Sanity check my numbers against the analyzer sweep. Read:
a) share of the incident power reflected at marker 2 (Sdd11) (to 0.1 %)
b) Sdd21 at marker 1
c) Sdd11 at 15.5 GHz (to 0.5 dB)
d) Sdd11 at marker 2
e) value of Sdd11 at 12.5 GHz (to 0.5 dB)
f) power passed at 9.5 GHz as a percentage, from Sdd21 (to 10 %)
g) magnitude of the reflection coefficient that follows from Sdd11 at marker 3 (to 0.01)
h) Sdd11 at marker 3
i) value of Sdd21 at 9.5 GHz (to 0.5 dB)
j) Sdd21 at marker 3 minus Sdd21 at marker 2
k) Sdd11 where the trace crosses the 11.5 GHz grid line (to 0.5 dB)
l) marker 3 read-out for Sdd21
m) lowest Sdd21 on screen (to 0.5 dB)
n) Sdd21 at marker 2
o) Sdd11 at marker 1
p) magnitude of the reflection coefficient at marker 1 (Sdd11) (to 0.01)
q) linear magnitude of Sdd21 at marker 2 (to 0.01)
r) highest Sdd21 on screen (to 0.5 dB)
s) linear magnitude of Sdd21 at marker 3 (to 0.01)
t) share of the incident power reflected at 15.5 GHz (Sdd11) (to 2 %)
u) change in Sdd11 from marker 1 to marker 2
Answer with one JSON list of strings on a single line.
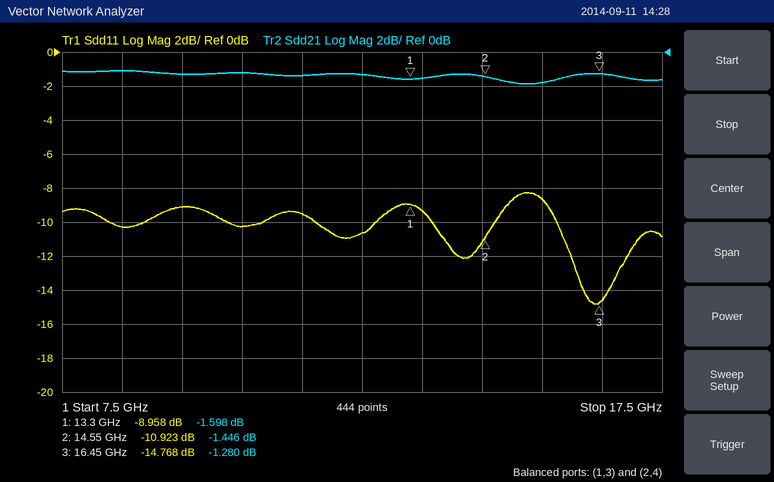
["8.1 %", "-1.598 dB", "-8.5 dB", "-10.923 dB", "-10.5 dB", "70 %", "0.18", "-14.768 dB", "-1.5 dB", "0.166 dB", "-9.5 dB", "-1.280 dB", "-2.0 dB", "-1.446 dB", "-8.958 dB", "0.36", "0.85", "-1.0 dB", "0.86", "14 %", "-1.965 dB"]
